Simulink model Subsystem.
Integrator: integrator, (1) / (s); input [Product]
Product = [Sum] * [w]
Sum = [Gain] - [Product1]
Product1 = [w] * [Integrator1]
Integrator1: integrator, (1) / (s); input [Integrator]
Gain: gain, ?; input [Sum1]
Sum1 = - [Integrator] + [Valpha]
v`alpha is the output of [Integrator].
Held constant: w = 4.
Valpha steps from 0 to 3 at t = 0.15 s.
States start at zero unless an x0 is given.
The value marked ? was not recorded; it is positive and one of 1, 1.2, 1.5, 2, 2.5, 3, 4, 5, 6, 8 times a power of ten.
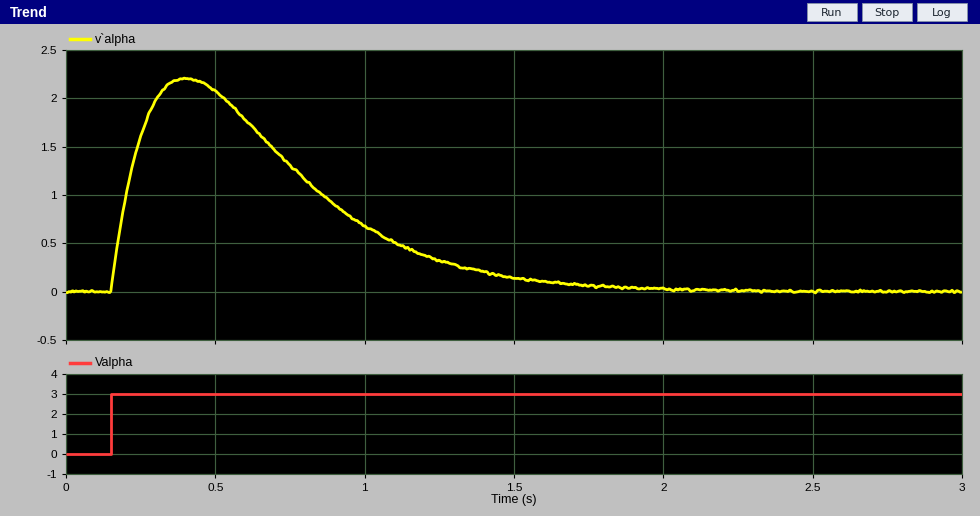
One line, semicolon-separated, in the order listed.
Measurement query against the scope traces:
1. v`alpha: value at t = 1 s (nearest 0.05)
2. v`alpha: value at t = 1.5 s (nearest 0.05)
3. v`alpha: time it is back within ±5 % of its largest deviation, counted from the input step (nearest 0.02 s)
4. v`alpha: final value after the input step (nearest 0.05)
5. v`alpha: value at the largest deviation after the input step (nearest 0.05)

0.70; 0.15; 1.44 s; 0.00; 2.20
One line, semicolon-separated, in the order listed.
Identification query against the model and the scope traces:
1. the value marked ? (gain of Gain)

2
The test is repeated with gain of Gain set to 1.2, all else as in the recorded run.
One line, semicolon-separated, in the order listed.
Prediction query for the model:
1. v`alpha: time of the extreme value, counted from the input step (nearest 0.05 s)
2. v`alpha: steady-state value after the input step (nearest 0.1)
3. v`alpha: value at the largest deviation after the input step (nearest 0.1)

0.30 s; 0.0; 1.8
